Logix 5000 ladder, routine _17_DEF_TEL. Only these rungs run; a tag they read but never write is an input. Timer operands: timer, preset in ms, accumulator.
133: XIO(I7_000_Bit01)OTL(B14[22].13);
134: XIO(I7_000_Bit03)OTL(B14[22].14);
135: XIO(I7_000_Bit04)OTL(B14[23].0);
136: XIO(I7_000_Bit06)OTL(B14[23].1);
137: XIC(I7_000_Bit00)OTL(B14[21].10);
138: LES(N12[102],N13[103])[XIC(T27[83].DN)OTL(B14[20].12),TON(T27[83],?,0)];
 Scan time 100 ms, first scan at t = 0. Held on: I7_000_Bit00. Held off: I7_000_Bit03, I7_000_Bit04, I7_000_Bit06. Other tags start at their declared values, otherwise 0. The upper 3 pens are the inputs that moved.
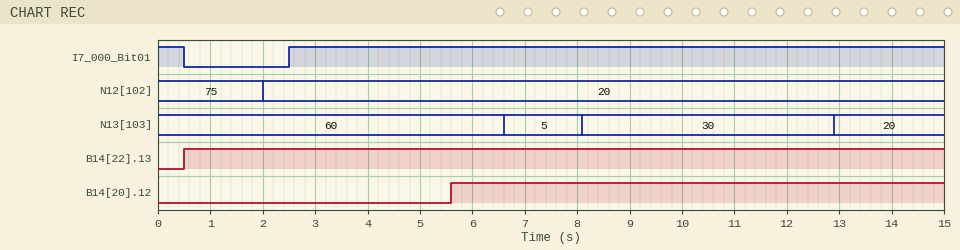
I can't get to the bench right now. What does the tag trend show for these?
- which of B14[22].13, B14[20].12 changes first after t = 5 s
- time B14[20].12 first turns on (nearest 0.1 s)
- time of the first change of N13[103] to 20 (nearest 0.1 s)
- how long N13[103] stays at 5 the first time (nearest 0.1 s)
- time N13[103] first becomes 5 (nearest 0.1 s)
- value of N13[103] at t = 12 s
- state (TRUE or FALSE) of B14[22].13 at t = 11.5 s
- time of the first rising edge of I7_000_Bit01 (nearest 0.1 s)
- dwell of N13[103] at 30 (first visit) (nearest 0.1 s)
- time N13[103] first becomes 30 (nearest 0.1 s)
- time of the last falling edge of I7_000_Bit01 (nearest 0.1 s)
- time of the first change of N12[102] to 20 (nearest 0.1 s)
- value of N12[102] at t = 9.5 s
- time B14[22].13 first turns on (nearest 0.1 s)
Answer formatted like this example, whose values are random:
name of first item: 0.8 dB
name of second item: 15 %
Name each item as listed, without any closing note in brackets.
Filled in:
which of B14[22].13, B14[20].12 changes first after t = 5 s: B14[20].12
time B14[20].12 first turns on: 5.6 s
time of the first change of N13[103] to 20: 12.9 s
how long N13[103] stays at 5 the first time: 1.5 s
time N13[103] first becomes 5: 6.6 s
value of N13[103] at t = 12 s: 30
state (TRUE or FALSE) of B14[22].13 at t = 11.5 s: TRUE
time of the first rising edge of I7_000_Bit01: 2.5 s
dwell of N13[103] at 30 (first visit): 4.8 s
time N13[103] first becomes 30: 8.1 s
time of the last falling edge of I7_000_Bit01: 0.5 s
time of the first change of N12[102] to 20: 2.0 s
value of N12[102] at t = 9.5 s: 20
time B14[22].13 first turns on: 0.5 s
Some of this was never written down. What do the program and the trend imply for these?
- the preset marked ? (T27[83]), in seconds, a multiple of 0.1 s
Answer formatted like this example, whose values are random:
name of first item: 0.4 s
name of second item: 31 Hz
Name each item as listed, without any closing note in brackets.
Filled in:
the preset marked ? (T27[83]), in seconds, a multiple of 0.1 s: 3.5 s
